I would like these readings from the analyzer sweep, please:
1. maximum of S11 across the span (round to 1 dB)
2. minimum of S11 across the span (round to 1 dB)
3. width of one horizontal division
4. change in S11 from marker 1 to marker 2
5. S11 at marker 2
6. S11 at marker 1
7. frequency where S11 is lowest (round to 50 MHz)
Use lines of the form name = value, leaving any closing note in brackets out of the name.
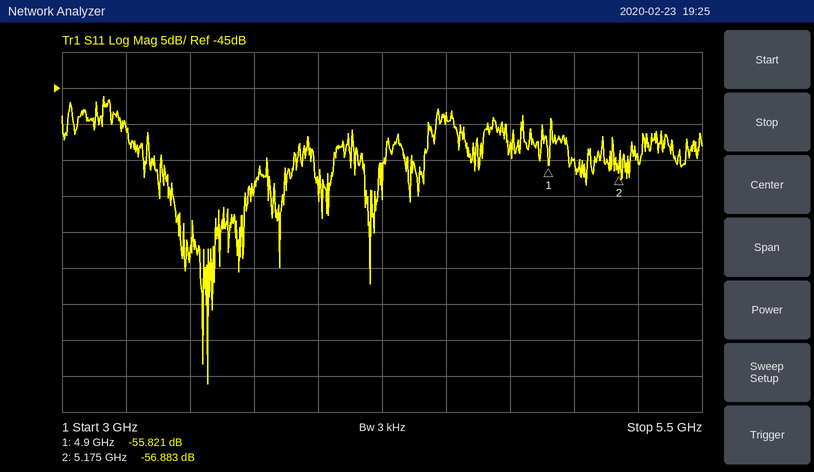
maximum of S11 across the span = -46 dB
minimum of S11 across the span = -86 dB
width of one horizontal division = 250 MHz
change in S11 from marker 1 to marker 2 = -1.062 dB
S11 at marker 2 = -56.883 dB
S11 at marker 1 = -55.821 dB
frequency where S11 is lowest = 3.55 GHz
